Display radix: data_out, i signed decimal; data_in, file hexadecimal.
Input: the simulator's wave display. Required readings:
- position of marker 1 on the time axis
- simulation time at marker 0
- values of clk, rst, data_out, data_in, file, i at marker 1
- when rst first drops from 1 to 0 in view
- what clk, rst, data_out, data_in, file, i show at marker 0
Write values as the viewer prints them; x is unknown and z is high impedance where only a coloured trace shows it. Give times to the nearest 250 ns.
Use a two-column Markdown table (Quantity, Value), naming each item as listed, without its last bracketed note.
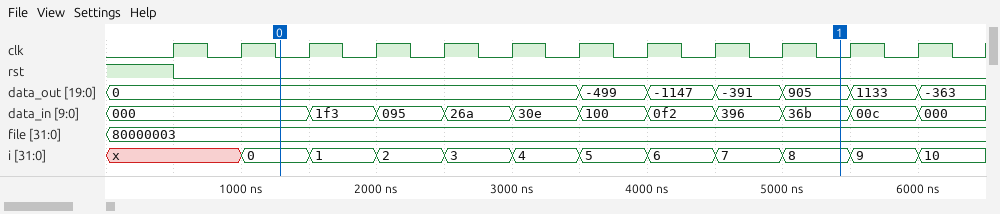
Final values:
| Quantity | Value |
|---|---|
| position of marker 1 on the time axis | 5500 ns |
| simulation time at marker 0 | 1250 ns |
| values of clk, rst, data_out, data_in, file, i at marker 1 | clk=0, rst=0, data_out=905, data_in=36b, file=80000003, i=8 |
| when rst first drops from 1 to 0 in view | 500 ns |
| what clk, rst, data_out, data_in, file, i show at marker 0 | clk=0, rst=0, data_out=0, data_in=000, file=80000003, i=0 |
